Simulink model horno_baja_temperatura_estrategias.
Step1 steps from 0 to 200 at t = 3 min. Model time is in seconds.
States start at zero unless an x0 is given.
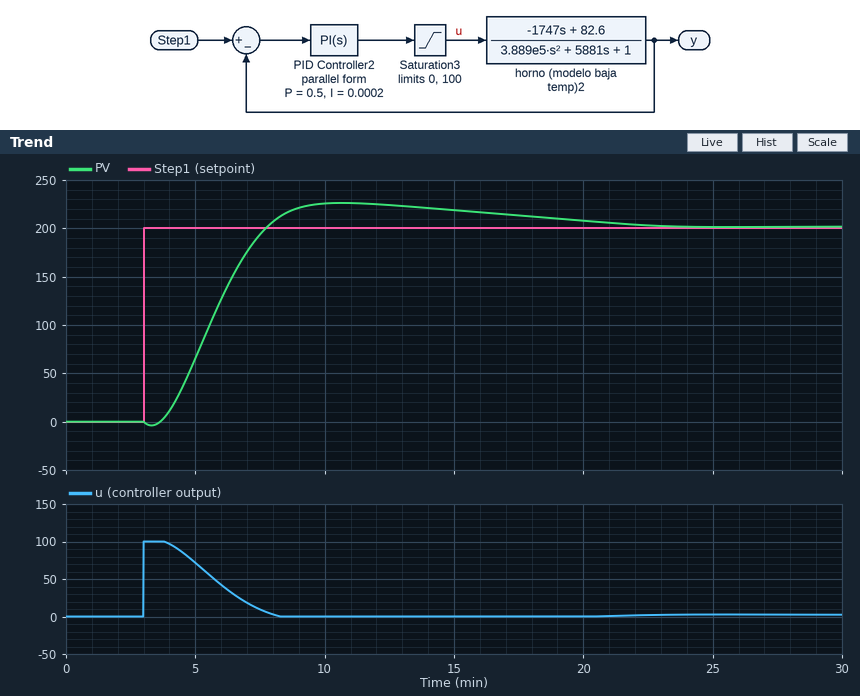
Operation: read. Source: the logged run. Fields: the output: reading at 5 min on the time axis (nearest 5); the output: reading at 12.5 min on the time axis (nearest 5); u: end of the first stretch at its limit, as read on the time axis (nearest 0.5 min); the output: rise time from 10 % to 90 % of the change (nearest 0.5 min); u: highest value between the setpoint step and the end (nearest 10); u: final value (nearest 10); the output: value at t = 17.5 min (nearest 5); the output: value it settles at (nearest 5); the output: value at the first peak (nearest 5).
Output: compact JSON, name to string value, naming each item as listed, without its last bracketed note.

{"the output: reading at 5 min on the time axis": "65", "the output: reading at 12.5 min on the time axis": "225", "u: end of the first stretch at its limit, as read on the time axis": "4.0 min", "the output: rise time from 10 % to 90 % of the change": "3.0 min", "u: highest value between the setpoint step and the end": "100", "u: final value": "0", "the output: value at t = 17.5 min": "215", "the output: value it settles at": "200", "the output: value at the first peak": "225"}
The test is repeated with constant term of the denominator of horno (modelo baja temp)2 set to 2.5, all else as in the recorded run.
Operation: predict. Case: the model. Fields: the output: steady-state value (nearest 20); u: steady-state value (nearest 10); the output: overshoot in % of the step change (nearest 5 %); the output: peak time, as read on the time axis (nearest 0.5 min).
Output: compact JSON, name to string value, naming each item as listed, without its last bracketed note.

{"the output: steady-state value": "200", "u: steady-state value": "10", "the output: overshoot in % of the step change": "10 %", "the output: peak time, as read on the time axis": "10.0 min"}
